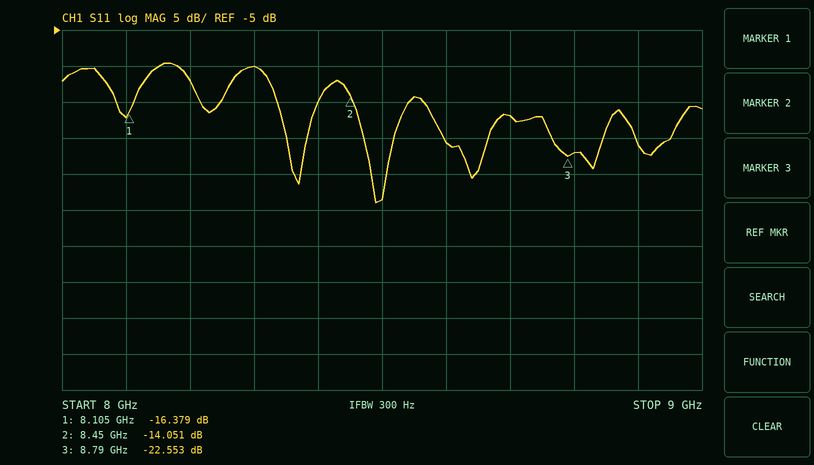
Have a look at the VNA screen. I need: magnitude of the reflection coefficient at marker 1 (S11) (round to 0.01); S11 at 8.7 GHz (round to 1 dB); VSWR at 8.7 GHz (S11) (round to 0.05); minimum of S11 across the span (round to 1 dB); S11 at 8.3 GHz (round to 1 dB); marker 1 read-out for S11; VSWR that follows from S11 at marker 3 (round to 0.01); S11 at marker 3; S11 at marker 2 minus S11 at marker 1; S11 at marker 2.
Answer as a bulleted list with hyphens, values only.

- 0.15
- -17 dB
- 1.35
- -29 dB
- -10 dB
- -16.379 dB
- 1.16
- -22.553 dB
- 2.328 dB
- -14.051 dB
